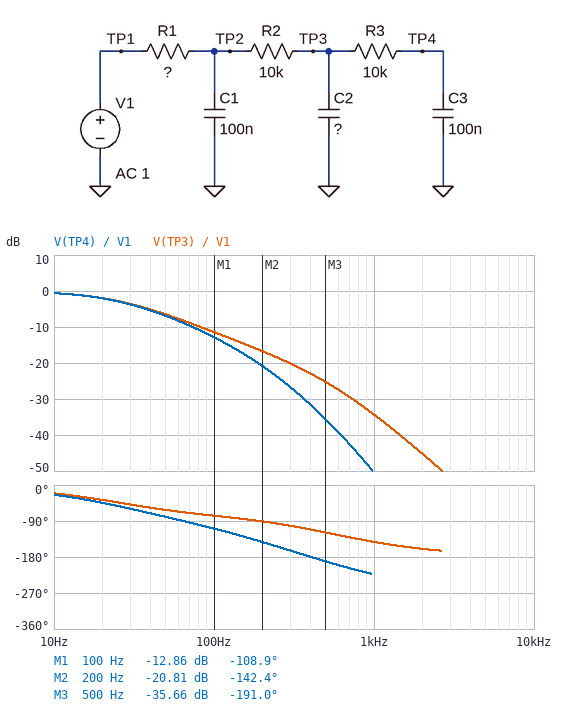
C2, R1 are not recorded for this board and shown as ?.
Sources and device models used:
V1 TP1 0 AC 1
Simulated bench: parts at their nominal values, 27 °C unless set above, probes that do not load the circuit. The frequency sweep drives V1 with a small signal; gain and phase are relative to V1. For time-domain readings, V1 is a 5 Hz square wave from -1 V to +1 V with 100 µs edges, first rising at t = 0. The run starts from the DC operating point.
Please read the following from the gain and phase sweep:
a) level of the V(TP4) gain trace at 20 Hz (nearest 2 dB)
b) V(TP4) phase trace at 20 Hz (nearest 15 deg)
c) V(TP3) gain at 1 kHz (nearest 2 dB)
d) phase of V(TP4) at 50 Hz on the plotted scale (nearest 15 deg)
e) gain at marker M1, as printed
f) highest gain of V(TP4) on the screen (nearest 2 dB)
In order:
-2 dB
-45 deg
-34 dB
-75 deg
-12.86 dB
0 dB
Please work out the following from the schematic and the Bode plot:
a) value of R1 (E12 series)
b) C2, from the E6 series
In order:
3.3 kΩ
330 nF
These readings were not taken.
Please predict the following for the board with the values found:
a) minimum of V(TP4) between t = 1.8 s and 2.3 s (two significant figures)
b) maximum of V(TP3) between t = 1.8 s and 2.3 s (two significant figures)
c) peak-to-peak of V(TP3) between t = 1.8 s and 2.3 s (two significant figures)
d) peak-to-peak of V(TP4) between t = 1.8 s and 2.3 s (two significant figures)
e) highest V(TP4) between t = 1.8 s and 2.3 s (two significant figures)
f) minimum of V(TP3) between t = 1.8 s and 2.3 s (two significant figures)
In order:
-1.0 V
1.0 V
2.0 V
2.0 V
1.0 V
-1.0 V
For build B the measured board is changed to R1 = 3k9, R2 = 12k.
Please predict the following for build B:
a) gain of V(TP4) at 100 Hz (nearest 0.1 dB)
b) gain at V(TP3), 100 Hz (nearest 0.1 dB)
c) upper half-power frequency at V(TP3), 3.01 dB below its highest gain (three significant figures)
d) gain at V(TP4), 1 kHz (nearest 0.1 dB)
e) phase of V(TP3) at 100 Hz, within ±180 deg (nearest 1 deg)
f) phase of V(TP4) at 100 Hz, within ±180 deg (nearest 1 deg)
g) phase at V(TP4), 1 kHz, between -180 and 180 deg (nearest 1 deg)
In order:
-14.3 dB
-12.9 dB
22.3 Hz
-53.0 dB
-81 deg
-113 deg
132 deg
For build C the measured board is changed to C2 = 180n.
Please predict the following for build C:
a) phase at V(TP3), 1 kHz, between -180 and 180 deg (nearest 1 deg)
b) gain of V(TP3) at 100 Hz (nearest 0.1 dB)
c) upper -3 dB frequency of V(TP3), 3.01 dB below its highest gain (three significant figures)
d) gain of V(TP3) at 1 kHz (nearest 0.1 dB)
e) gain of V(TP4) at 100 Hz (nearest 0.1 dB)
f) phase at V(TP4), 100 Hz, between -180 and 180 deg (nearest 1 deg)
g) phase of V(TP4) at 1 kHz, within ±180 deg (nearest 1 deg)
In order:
-138 deg
-8.3 dB
39.0 Hz
-29.2 dB
-9.7 dB
-98 deg
141 deg
